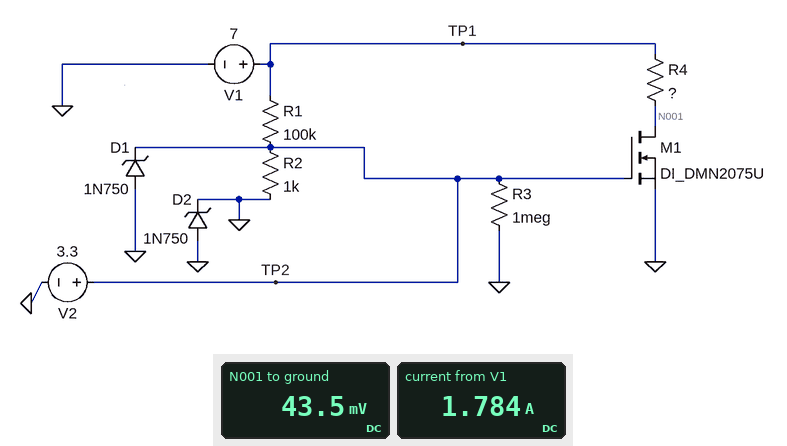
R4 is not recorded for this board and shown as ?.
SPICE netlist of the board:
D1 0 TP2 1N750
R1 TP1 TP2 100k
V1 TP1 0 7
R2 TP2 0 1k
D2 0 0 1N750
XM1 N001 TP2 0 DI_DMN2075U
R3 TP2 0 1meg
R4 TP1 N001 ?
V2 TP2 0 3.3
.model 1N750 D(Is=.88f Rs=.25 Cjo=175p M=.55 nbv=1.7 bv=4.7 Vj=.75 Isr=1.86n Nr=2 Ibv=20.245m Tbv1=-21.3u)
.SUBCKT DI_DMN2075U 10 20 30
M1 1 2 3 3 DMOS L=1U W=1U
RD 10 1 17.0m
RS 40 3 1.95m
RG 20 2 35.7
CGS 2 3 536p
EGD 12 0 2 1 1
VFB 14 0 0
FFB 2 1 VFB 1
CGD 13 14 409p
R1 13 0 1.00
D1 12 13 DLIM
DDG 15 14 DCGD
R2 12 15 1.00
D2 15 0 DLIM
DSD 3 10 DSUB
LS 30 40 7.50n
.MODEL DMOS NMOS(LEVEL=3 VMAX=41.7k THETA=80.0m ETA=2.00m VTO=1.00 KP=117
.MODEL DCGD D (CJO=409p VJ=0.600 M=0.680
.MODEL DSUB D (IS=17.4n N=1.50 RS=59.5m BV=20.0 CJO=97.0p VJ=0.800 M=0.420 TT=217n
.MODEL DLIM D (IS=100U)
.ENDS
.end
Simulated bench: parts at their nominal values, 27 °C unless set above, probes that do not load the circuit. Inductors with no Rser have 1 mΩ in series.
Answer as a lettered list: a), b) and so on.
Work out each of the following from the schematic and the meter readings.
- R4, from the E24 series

a) 3.9 Ω
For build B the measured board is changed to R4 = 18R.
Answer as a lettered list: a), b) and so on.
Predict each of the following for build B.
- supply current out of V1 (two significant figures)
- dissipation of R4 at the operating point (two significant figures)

a) 390 mA
b) 2.7 W
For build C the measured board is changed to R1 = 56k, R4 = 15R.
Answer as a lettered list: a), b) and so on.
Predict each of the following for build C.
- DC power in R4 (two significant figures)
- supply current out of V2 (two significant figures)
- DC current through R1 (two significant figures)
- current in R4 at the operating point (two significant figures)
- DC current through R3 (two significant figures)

a) 3.3 W
b) 3.2 mA
c) 66 µA
d) 470 mA
e) 3.3 µA
